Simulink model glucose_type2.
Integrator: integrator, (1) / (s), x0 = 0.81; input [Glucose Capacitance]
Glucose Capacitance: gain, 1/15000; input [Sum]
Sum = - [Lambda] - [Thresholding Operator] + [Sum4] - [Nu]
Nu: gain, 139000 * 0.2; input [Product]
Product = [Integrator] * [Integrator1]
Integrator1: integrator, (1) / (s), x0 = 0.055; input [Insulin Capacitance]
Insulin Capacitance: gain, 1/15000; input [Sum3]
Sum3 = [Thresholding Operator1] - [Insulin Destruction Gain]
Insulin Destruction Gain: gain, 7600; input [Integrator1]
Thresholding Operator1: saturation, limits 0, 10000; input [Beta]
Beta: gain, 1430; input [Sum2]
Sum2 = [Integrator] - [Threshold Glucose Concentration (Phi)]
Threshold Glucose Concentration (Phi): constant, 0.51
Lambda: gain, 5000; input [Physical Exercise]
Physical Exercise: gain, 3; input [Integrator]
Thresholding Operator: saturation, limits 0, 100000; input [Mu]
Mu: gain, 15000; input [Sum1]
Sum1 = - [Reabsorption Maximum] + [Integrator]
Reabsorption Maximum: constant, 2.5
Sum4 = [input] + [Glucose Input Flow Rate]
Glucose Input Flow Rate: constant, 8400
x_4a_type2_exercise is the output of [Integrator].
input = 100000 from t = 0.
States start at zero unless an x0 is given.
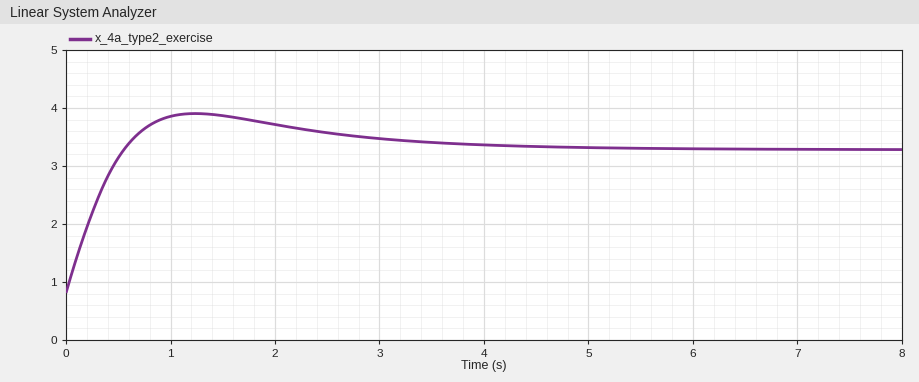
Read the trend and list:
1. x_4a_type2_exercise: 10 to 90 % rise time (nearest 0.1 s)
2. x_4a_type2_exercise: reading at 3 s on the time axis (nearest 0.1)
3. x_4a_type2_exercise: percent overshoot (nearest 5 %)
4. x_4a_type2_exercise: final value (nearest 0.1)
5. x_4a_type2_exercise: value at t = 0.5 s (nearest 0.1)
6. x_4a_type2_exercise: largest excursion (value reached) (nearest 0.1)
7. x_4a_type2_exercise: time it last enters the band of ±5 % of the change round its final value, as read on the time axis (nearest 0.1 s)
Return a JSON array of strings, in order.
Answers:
["0.4 s", "3.5", "25 %", "3.3", "3.1", "3.9", "3.5 s"]
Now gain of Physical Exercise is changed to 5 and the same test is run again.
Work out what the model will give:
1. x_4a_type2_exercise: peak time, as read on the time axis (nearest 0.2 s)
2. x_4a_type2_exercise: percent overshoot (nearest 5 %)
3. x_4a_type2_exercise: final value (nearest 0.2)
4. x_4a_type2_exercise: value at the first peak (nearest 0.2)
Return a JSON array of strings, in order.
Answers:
["1.2 s", "20 %", "2.8", "3.2"]
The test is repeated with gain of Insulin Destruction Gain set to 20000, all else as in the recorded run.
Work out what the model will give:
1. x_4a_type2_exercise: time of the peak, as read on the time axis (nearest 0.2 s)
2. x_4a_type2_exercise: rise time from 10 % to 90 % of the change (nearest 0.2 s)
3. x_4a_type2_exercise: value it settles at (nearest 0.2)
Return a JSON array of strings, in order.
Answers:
["1.6 s", "0.6 s", "4.0"]
